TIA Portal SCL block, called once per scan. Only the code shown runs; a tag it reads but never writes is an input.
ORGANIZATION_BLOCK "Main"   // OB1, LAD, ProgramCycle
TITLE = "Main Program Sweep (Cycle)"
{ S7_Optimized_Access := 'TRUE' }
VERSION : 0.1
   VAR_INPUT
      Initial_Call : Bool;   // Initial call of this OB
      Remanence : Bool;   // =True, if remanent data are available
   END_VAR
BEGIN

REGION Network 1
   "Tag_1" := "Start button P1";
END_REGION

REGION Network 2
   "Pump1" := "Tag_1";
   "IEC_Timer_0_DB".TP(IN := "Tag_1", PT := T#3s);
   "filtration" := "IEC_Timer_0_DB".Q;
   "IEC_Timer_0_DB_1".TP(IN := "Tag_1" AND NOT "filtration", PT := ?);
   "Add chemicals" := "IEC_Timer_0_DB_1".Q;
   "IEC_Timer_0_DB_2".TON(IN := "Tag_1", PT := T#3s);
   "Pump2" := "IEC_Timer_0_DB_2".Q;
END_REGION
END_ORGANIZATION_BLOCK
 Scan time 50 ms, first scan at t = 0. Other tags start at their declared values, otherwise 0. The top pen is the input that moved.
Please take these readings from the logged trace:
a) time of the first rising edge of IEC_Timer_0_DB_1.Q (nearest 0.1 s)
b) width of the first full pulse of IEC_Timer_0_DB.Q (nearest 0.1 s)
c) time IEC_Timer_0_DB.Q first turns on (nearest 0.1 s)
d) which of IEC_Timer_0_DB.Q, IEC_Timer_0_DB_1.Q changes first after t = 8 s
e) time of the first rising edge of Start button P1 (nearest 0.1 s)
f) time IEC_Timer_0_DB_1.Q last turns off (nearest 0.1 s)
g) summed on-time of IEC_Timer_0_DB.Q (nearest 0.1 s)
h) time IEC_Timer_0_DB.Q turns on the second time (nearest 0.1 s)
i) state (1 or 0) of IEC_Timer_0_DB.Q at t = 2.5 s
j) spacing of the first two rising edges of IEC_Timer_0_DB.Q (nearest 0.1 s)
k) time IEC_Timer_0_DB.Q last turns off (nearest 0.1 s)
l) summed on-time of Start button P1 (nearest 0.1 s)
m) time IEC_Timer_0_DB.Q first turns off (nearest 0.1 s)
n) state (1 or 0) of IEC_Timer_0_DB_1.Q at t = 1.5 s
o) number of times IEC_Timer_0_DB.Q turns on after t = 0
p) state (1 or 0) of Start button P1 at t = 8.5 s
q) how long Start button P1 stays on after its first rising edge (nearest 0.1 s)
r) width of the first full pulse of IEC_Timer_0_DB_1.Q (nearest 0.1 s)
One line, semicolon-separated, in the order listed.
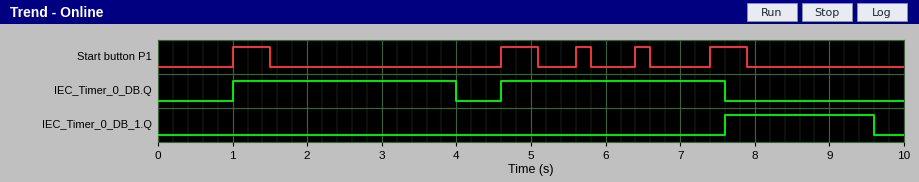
7.6 s; 3.0 s; 1.0 s; IEC_Timer_0_DB_1.Q; 1.0 s; 9.6 s; 6.0 s; 4.6 s; 1; 3.6 s; 7.6 s; 1.9 s; 4.0 s; 0; 2; 0; 0.5 s; 2.0 s
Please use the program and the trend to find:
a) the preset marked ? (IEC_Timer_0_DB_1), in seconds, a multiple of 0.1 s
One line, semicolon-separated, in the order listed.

2.0 s
